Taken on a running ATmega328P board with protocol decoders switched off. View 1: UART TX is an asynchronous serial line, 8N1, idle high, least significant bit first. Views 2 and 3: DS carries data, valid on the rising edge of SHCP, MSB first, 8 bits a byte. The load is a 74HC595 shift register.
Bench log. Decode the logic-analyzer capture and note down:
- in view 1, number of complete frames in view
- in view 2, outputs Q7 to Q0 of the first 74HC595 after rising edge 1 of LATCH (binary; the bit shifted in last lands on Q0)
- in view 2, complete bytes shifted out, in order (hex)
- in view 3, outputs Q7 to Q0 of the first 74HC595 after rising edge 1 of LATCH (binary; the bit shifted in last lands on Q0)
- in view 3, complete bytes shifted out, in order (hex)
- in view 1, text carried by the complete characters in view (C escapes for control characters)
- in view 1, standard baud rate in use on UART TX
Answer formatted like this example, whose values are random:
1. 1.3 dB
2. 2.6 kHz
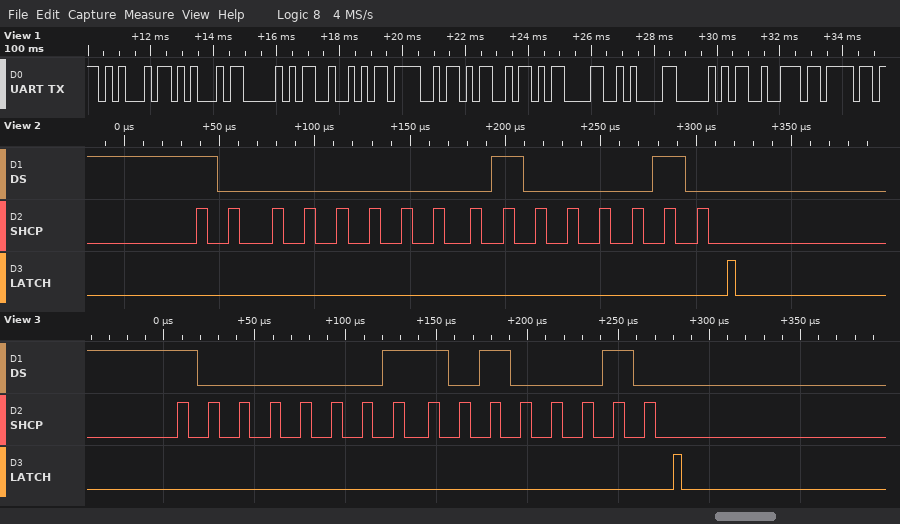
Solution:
1. 11
2. 01000010
3. 0x80 0x42
4. 10100010
5. 81 A2
6. "EEPROM\r\nPro"
7. 4800 baud
